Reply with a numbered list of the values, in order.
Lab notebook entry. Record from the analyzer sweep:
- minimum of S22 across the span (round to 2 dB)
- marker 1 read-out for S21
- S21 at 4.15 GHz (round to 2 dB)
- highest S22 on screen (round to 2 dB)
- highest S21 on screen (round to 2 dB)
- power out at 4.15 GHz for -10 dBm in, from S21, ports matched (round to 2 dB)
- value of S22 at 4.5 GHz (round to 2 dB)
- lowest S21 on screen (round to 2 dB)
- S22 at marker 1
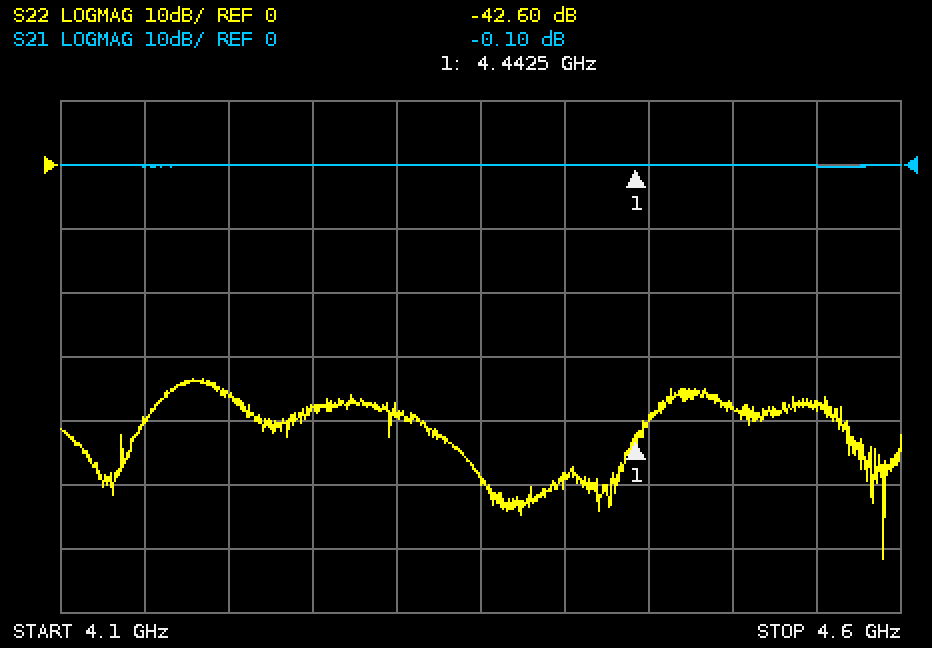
1. -62 dB
2. -0.10 dB
3. 0 dB
4. -34 dB
5. 0 dB
6. -10 dBm
7. -38 dB
8. 0 dB
9. -42.60 dB
